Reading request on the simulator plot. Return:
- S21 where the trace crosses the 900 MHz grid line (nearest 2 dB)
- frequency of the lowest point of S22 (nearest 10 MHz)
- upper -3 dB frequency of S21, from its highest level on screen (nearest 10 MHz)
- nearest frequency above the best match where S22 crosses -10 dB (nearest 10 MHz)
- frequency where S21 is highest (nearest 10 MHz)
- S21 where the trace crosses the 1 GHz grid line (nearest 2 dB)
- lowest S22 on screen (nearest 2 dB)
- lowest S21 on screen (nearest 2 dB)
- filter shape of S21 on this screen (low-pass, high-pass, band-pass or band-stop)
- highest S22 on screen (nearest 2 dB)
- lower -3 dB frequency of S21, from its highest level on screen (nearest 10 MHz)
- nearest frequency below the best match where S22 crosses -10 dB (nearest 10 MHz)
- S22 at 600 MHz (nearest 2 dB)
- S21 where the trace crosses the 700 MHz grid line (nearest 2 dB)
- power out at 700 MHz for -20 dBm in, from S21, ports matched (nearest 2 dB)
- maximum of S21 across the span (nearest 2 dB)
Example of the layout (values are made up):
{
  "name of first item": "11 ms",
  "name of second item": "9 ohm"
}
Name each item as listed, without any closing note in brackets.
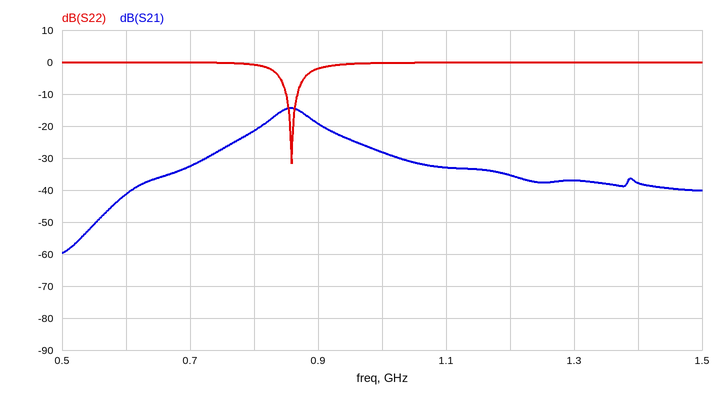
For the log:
{
  "S21 where the trace crosses the 900 MHz grid line": "-20 dB",
  "frequency of the lowest point of S22": "860 MHz",
  "upper -3 dB frequency of S21, from its highest level on screen": "890 MHz",
  "nearest frequency above the best match where S22 crosses -10 dB": "870 MHz",
  "frequency where S21 is highest": "860 MHz",
  "S21 where the trace crosses the 1 GHz grid line": "-28 dB",
  "lowest S22 on screen": "-32 dB",
  "lowest S21 on screen": "-60 dB",
  "filter shape of S21 on this screen": "band-pass",
  "highest S22 on screen": "0 dB",
  "lower -3 dB frequency of S21, from its highest level on screen": "830 MHz",
  "nearest frequency below the best match where S22 crosses -10 dB": "850 MHz",
  "S22 at 600 MHz": "0 dB",
  "S21 where the trace crosses the 700 MHz grid line": "-32 dB",
  "power out at 700 MHz for -20 dBm in, from S21, ports matched": "-52 dBm",
  "maximum of S21 across the span": "-14 dB"
}
